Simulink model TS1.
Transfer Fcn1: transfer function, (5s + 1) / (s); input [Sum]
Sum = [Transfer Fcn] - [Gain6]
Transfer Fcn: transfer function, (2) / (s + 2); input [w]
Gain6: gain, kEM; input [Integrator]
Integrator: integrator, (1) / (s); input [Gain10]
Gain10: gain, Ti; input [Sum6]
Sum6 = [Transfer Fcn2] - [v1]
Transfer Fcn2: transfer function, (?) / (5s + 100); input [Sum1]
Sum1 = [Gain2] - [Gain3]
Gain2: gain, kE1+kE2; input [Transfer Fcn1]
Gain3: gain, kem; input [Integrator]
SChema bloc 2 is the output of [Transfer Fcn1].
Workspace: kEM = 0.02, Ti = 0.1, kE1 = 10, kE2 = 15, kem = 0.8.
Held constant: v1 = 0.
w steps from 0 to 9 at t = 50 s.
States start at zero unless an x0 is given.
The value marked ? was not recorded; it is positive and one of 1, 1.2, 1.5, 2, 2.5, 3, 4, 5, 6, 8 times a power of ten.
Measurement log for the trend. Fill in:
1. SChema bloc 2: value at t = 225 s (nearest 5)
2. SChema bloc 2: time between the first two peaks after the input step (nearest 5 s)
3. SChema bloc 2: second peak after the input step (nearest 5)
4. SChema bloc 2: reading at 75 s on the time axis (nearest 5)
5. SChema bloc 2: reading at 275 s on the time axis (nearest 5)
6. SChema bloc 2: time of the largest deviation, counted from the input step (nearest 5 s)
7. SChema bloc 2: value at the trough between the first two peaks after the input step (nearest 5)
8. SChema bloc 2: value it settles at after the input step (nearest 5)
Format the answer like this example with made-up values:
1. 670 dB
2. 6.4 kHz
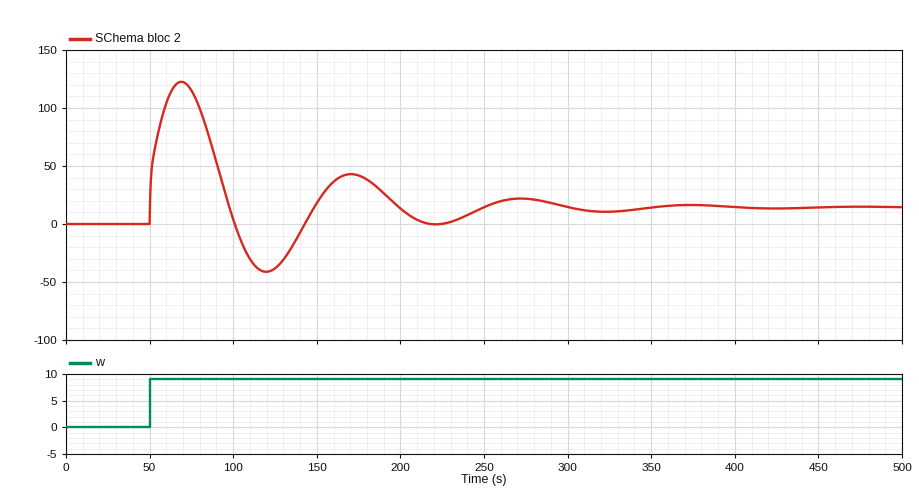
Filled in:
1. 0
2. 100 s
3. 45
4. 115
5. 20
6. 20 s
7. -40
8. 15
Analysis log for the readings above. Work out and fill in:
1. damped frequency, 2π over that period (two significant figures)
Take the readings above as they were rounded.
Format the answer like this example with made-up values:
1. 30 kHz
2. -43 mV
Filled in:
1. 0.063 rad/s
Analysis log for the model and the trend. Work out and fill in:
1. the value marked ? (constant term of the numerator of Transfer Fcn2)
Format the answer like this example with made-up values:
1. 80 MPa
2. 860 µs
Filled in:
1. 8
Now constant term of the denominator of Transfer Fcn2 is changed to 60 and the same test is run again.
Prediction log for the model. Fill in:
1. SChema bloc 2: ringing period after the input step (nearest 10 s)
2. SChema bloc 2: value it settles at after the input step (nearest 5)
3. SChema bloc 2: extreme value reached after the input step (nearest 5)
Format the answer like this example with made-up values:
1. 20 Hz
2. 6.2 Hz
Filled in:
1. 80 s
2. 15
3. 95
